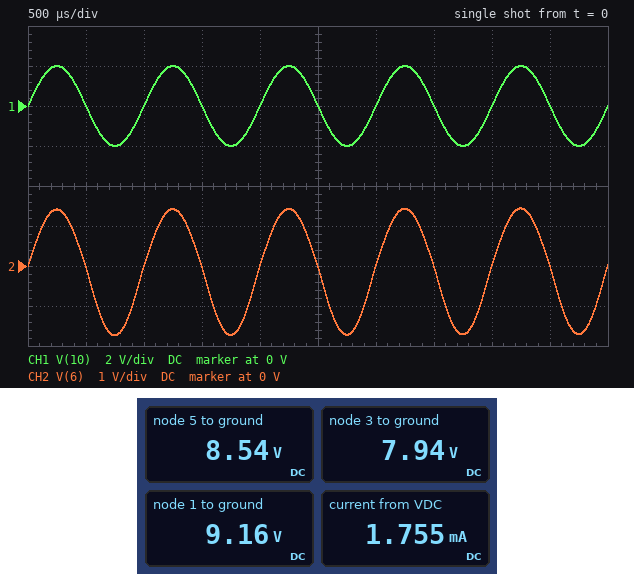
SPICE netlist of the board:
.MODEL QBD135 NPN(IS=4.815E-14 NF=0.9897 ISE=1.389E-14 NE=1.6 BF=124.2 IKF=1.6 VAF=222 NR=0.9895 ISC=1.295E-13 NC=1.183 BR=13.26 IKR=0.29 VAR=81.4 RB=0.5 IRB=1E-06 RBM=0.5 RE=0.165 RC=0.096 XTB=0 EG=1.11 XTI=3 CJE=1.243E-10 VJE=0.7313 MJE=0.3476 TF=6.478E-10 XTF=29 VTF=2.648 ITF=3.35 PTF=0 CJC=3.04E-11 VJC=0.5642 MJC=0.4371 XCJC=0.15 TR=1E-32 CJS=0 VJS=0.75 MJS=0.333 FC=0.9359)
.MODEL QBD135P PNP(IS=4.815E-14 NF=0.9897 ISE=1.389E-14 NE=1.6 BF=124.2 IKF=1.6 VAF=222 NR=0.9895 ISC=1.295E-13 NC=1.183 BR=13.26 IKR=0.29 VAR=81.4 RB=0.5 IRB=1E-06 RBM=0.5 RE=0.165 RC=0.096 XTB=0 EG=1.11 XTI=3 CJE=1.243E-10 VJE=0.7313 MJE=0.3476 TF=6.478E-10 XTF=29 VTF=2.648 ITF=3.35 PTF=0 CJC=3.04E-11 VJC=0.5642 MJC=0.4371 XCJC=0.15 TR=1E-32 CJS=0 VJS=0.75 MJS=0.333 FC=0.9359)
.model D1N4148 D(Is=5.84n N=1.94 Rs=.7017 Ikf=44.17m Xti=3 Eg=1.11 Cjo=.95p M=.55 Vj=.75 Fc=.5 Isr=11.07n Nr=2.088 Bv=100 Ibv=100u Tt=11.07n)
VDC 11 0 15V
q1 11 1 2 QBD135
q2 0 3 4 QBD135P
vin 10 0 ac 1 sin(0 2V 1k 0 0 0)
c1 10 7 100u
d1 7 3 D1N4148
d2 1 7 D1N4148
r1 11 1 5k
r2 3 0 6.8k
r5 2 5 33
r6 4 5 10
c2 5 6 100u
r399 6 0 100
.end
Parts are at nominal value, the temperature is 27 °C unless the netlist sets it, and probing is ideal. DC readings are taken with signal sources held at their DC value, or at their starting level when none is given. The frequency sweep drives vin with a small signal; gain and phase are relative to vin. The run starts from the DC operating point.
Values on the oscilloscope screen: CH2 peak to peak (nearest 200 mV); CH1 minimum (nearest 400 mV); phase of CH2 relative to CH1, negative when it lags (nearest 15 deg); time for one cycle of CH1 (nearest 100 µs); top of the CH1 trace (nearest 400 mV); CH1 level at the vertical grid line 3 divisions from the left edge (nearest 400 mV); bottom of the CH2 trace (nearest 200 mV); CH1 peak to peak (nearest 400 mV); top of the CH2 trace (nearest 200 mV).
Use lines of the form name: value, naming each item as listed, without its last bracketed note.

CH2 peak to peak: 3.2 V
CH1 minimum: -2.0 V
phase of CH2 relative to CH1, negative when it lags: 0 deg
time for one cycle of CH1: 1.0 ms
top of the CH1 trace: 2.0 V
CH1 level at the vertical grid line 3 divisions from the left edge: 0 V
bottom of the CH2 trace: -1.8 V
CH1 peak to peak: 4.0 V
top of the CH2 trace: 1.4 V
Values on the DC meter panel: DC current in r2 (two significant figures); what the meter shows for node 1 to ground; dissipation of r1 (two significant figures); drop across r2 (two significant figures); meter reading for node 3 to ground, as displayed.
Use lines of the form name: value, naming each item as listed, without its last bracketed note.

DC current in r2: 1.2 mA
what the meter shows for node 1 to ground: 9.16 V
dissipation of r1: 6.8 mW
drop across r2: 7.9 V
meter reading for node 3 to ground, as displayed: 7.94 V
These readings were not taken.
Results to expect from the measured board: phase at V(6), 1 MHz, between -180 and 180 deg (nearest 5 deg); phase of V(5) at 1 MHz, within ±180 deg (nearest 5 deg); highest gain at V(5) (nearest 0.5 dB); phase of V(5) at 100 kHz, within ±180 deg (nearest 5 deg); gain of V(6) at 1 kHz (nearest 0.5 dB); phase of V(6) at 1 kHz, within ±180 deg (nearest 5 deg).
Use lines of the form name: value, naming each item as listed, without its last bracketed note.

phase at V(6), 1 MHz, between -180 and 180 deg: 0 deg
phase of V(5) at 1 MHz, within ±180 deg: 0 deg
highest gain at V(5): -0.5 dB
phase of V(5) at 100 kHz, within ±180 deg: 0 deg
gain of V(6) at 1 kHz: -2.5 dB
phase of V(6) at 1 kHz, within ±180 deg: 0 deg
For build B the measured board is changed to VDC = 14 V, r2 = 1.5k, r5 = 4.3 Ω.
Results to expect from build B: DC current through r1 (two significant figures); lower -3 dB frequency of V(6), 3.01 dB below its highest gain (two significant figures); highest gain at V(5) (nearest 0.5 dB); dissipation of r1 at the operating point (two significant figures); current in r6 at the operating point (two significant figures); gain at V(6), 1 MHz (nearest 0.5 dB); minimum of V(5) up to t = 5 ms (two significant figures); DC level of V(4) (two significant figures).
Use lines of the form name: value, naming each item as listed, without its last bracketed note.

DC current through r1: 2.0 mA
lower -3 dB frequency of V(6), 3.01 dB below its highest gain: 16 Hz
highest gain at V(5): -0.5 dB
dissipation of r1 at the operating point: 19 mW
current in r6 at the operating point: 1.9 mA
gain at V(6), 1 MHz: -1.0 dB
minimum of V(5) up to t = 5 ms: 1.9 V
DC level of V(4): 3.6 V
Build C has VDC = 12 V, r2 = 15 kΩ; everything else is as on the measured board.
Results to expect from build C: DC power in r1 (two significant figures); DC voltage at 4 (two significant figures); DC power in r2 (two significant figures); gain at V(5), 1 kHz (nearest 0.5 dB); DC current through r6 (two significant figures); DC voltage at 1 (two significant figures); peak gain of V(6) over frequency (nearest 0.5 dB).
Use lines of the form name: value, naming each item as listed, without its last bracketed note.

DC power in r1: 1.5 mW
DC voltage at 4: 8.7 V
DC power in r2: 4.4 mW
gain at V(5), 1 kHz: -6.0 dB
DC current through r6: 150 µA
DC voltage at 1: 9.3 V
peak gain of V(6) over frequency: -1.5 dB
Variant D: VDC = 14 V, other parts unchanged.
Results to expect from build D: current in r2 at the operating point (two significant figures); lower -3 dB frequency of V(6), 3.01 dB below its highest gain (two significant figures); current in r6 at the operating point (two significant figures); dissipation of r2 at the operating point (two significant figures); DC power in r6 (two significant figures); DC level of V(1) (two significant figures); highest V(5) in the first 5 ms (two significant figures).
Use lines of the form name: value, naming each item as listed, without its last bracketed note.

current in r2 at the operating point: 1.1 mA
lower -3 dB frequency of V(6), 3.01 dB below its highest gain: 19 Hz
current in r6 at the operating point: 530 µA
dissipation of r2 at the operating point: 8.0 mW
DC power in r6: 2.8 µW
DC level of V(1): 8.6 V
highest V(5) in the first 5 ms: 9.4 V
